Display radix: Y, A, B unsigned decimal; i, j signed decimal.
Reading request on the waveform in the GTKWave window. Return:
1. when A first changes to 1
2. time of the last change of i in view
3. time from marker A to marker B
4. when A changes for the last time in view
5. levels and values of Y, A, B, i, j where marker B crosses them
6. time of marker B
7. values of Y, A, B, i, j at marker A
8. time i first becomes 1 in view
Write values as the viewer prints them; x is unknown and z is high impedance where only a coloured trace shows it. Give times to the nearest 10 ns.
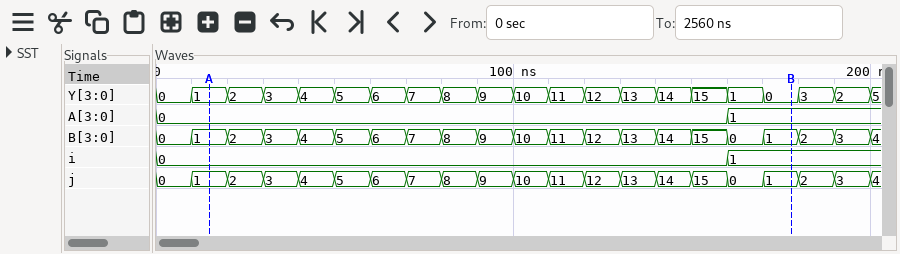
160 ns
160 ns
160 ns
160 ns
Y=0, A=1, B=1, i=1, j=1
180 ns
Y=1, A=0, B=1, i=0, j=1
160 ns
